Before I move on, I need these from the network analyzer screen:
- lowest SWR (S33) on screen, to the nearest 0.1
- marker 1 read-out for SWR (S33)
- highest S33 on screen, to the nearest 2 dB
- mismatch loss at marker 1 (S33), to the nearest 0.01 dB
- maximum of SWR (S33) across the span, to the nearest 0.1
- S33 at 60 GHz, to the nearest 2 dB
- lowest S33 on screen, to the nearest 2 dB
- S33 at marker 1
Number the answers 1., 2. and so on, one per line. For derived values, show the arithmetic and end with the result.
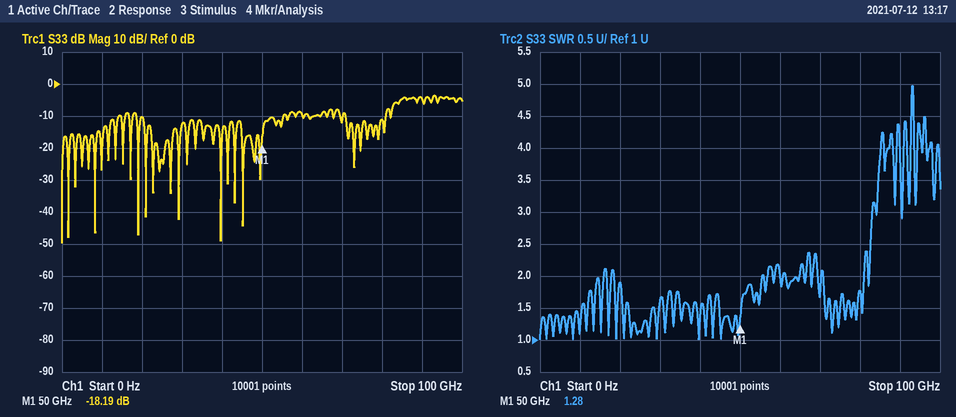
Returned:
1. 1.0
2. 1.28
3. -4 dB
4. −10 log10(1 − 10^(-18.19/10)) ≈ 0.07 dB
5. 5.0
6. -10 dB
7. -50 dB
8. -18.19 dB
